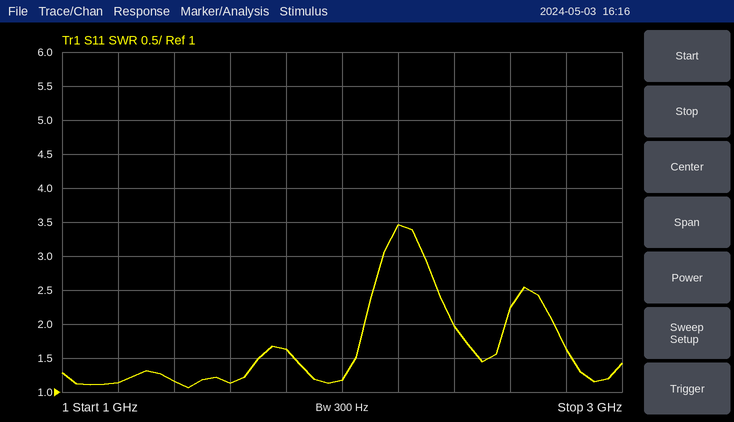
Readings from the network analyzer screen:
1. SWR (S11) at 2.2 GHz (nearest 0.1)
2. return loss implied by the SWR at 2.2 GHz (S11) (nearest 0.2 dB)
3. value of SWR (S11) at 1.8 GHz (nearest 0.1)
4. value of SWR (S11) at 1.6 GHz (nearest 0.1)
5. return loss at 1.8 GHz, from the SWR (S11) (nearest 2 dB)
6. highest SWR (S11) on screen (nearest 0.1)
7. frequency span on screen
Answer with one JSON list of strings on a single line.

["3.5", "5.2 dB", "1.6", "1.1", "12 dB", "3.5", "2 GHz"]
